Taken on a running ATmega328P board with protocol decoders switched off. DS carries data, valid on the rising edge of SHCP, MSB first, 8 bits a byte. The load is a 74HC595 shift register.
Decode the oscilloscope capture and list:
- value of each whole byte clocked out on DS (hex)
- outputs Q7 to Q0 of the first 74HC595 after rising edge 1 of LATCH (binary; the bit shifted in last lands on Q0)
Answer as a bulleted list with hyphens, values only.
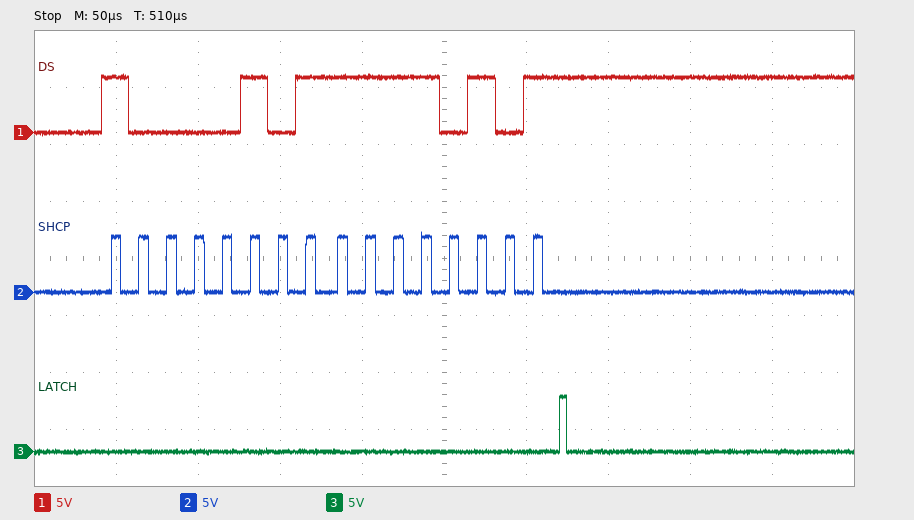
- 0x85 0xF5
- 11110101
